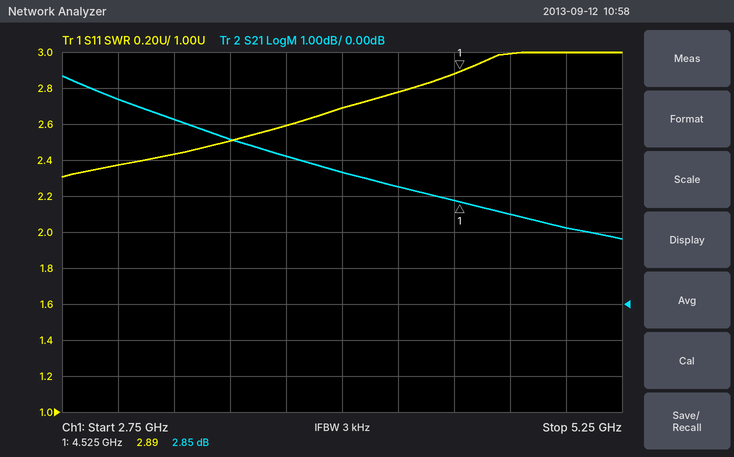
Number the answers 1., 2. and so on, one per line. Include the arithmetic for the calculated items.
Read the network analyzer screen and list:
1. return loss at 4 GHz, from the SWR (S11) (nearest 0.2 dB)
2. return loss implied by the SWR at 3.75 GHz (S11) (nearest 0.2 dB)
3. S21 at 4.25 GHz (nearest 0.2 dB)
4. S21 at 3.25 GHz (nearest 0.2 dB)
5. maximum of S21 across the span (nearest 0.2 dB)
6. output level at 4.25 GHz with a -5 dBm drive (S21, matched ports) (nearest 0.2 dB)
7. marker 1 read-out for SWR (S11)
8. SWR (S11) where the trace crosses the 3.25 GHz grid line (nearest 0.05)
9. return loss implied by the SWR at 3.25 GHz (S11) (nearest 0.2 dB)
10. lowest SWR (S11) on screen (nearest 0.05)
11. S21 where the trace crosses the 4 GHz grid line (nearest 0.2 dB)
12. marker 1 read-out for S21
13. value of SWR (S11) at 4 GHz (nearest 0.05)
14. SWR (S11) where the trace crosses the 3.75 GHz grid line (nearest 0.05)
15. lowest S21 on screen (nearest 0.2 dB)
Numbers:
1. −20 log10((2.7 − 1)/(2.7 + 1)) ≈ 6.8 dB
2. −20 log10((2.6 − 1)/(2.6 + 1)) ≈ 7.0 dB
3. 3.2 dB
4. 5.2 dB
5. 6.4 dB
6. -5 dBm + (3.2 dB) = -1.8 dBm
7. 2.89
8. 2.45
9. −20 log10((2.45 − 1)/(2.45 + 1)) ≈ 7.53 dB, so 7.6 dB to the nearest 0.2 dB
10. 2.30
11. 3.6 dB
12. 2.85 dB
13. 2.70
14. 2.60
15. 1.8 dB
